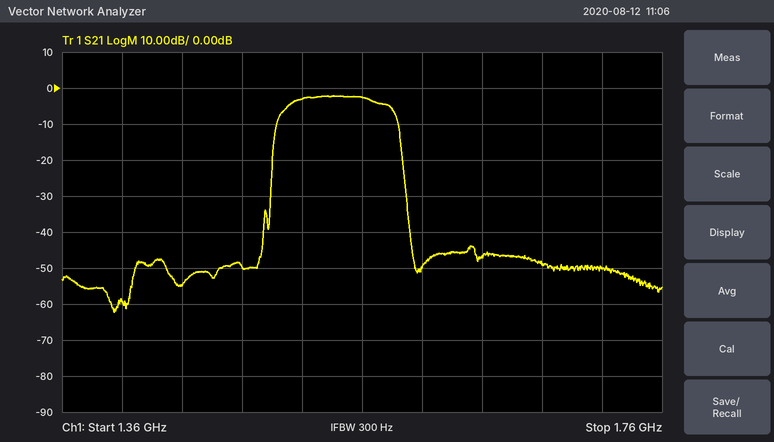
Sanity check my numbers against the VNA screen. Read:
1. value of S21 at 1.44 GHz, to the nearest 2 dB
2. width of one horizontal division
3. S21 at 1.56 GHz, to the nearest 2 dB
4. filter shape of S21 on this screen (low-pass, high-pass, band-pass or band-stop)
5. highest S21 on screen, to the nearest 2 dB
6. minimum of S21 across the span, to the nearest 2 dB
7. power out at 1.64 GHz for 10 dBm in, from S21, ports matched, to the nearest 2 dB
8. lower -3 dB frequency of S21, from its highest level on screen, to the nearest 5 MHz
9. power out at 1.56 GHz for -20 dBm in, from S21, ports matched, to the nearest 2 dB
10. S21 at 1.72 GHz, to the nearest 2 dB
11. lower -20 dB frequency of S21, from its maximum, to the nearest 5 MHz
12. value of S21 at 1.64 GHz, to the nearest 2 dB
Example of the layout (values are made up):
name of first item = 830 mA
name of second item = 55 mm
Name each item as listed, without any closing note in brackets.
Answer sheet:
value of S21 at 1.44 GHz, to the nearest 2 dB = -54 dB
width of one horizontal division = 40 MHz
S21 at 1.56 GHz, to the nearest 2 dB = -2 dB
filter shape of S21 on this screen = band-pass
highest S21 on screen, to the nearest 2 dB = -2 dB
minimum of S21 across the span, to the nearest 2 dB = -62 dB
power out at 1.64 GHz for 10 dBm in, from S21, ports matched, to the nearest 2 dB = -36 dBm
lower -3 dB frequency of S21, from its highest level on screen, to the nearest 5 MHz = 1.510 GHz
power out at 1.56 GHz for -20 dBm in, from S21, ports matched, to the nearest 2 dB = -22 dBm
S21 at 1.72 GHz, to the nearest 2 dB = -50 dB
lower -20 dB frequency of S21, from its maximum, to the nearest 5 MHz = 1.500 GHz
value of S21 at 1.64 GHz, to the nearest 2 dB = -46 dB
